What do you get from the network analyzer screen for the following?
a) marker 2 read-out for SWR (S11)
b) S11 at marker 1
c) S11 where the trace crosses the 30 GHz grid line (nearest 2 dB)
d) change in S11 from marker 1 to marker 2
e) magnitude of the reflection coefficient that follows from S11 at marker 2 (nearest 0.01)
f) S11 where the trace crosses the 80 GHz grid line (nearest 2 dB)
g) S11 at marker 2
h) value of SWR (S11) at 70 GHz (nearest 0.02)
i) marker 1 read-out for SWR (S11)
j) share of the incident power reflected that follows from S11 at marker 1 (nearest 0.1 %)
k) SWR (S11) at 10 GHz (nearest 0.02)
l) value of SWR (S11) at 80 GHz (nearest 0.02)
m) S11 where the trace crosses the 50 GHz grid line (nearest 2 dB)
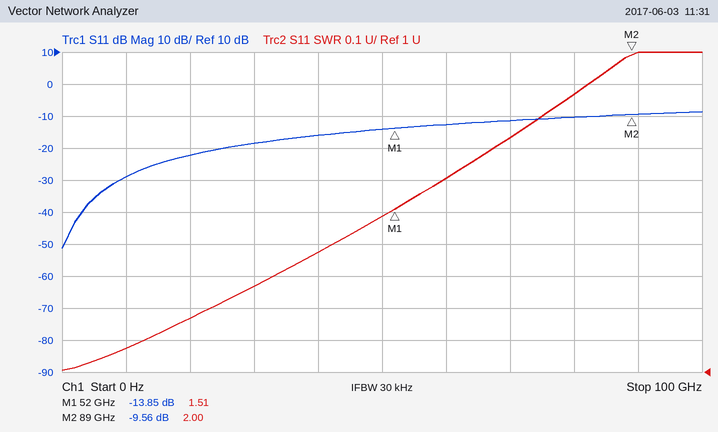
2.00
-13.85 dB
-18 dB
4.29 dB
0.33
-10 dB
-9.56 dB
1.74
1.51
4.1 %
1.08
1.86
-14 dB
